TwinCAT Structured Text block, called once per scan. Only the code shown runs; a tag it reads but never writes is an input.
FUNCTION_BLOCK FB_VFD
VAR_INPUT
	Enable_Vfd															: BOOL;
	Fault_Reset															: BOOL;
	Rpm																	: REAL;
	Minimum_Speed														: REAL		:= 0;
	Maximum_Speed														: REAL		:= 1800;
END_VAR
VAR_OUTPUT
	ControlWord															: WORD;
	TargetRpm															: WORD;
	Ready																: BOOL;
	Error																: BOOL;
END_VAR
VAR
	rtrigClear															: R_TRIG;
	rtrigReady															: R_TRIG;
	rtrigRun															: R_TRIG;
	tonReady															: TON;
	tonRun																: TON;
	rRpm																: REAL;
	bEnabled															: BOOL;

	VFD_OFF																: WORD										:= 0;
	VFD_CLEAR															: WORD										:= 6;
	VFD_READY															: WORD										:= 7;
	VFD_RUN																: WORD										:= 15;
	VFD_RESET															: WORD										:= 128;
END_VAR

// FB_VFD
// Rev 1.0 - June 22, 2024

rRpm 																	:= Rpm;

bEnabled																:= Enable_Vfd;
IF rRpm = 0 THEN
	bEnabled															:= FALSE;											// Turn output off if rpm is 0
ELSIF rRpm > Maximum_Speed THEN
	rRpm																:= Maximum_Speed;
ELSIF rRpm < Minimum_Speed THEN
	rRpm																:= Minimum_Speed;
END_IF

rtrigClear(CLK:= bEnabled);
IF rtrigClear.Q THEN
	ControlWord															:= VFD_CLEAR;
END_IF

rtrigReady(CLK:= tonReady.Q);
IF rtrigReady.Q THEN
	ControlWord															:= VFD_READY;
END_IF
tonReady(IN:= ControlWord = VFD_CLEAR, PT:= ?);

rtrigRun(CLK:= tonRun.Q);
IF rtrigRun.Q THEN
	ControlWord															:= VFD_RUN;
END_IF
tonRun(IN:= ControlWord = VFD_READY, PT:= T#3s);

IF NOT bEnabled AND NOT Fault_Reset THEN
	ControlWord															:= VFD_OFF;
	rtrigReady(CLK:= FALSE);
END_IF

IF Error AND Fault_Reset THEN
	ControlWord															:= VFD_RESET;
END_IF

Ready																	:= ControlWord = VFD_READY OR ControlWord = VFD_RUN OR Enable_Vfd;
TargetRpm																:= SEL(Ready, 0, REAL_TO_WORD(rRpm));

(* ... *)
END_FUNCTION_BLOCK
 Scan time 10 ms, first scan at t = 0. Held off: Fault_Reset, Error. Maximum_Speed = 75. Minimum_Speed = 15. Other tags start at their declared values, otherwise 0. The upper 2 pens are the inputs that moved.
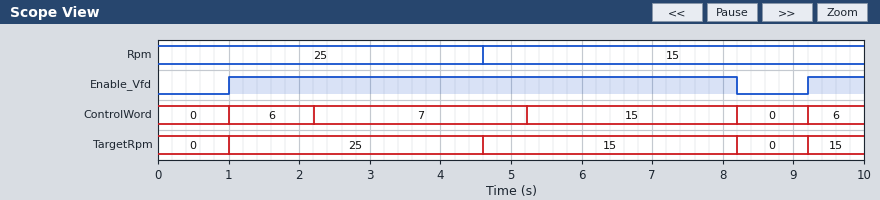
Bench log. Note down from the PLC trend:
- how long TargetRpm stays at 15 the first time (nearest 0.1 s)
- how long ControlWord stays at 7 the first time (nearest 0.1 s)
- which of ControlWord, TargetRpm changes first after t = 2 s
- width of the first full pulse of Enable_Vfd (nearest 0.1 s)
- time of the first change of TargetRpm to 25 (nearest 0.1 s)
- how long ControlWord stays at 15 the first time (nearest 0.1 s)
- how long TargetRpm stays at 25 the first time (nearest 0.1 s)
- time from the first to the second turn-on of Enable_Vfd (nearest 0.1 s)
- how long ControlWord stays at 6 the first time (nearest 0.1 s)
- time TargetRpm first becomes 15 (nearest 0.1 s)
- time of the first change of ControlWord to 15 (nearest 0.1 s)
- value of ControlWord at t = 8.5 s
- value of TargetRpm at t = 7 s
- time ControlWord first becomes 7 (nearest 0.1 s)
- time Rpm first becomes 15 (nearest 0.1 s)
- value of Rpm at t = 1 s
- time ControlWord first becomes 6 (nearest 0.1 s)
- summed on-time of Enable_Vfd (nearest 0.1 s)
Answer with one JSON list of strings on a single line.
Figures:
["3.6 s", "3.0 s", "ControlWord", "7.2 s", "1.0 s", "3.0 s", "3.6 s", "8.2 s", "1.2 s", "4.6 s", "5.2 s", "0", "15", "2.2 s", "4.6 s", "25", "1.0 s", "8.0 s"]
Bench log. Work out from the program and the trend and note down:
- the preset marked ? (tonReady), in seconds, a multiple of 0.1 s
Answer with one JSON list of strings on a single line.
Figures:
["1.2 s"]
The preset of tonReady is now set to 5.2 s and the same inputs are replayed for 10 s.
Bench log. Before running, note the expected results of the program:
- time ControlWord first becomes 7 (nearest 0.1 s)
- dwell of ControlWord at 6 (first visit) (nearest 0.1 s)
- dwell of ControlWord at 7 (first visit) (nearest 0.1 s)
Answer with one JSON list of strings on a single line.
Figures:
["6.2 s", "5.2 s", "2.0 s"]
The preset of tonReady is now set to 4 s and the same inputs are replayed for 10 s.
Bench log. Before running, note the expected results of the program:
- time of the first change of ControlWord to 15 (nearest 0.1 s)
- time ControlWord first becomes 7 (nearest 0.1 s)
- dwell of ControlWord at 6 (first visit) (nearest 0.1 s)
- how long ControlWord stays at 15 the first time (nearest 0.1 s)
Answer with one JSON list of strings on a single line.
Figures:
["8.0 s", "5.0 s", "4.0 s", "0.2 s"]
